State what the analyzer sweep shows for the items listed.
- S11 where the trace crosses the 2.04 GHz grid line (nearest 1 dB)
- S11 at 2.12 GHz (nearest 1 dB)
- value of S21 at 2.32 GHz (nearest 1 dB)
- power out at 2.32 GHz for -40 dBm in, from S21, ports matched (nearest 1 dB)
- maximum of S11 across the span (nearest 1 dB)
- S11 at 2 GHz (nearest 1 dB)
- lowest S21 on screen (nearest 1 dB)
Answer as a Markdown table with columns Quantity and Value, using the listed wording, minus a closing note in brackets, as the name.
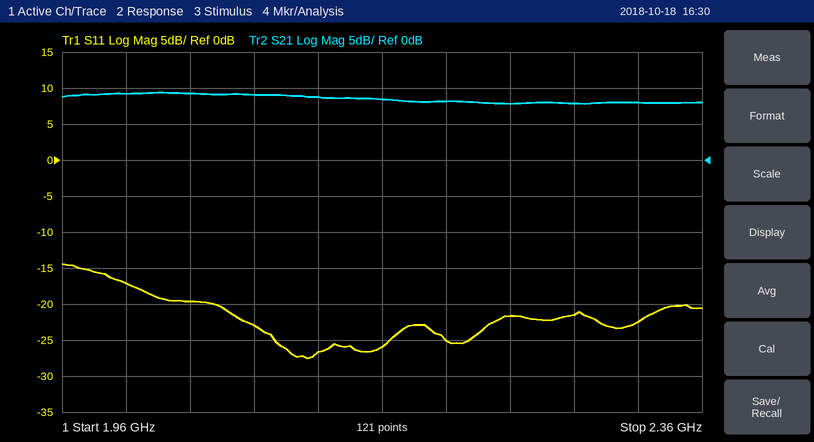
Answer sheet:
| Quantity | Value |
|---|---|
| S11 where the trace crosses the 2.04 GHz grid line | -20 dB |
| S11 at 2.12 GHz | -27 dB |
| value of S21 at 2.32 GHz | 8 dB |
| power out at 2.32 GHz for -40 dBm in, from S21, ports matched | -32 dBm |
| maximum of S11 across the span | -14 dB |
| S11 at 2 GHz | -17 dB |
| lowest S21 on screen | 8 dB |
